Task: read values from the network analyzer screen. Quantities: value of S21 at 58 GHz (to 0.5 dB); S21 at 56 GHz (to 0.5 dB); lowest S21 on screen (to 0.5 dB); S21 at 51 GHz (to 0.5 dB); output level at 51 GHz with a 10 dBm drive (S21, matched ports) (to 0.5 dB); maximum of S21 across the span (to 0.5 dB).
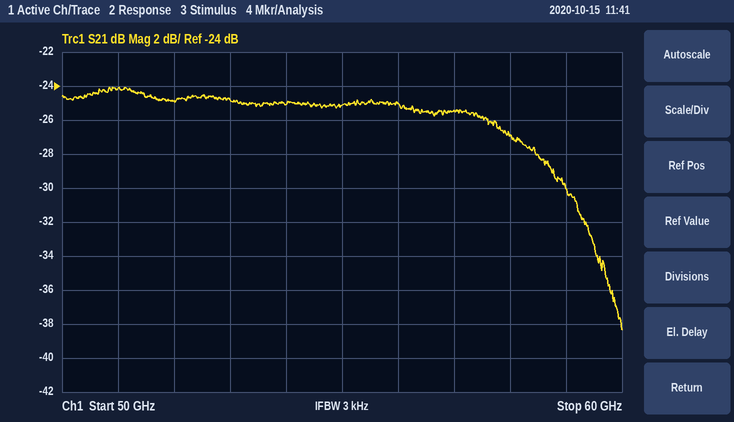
-27.0 dB
-25.0 dB
-38.5 dB
-24.0 dB
-14.0 dBm
-24.0 dB
